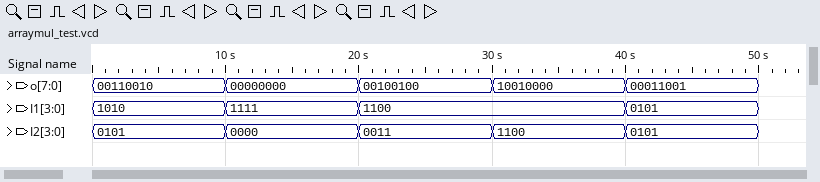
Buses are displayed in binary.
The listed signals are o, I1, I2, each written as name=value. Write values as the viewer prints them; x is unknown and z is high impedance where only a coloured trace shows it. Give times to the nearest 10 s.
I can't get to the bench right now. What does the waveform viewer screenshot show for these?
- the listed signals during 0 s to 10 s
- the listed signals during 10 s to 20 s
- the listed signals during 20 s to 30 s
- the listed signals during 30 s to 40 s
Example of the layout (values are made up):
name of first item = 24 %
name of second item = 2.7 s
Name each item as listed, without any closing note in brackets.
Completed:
the listed signals during 0 s to 10 s = o=00110010, I1=1010, I2=0101
the listed signals during 10 s to 20 s = o=00000000, I1=1111, I2=0000
the listed signals during 20 s to 30 s = o=00100100, I1=1100, I2=0011
the listed signals during 30 s to 40 s = o=10010000, I1=1100, I2=1100
